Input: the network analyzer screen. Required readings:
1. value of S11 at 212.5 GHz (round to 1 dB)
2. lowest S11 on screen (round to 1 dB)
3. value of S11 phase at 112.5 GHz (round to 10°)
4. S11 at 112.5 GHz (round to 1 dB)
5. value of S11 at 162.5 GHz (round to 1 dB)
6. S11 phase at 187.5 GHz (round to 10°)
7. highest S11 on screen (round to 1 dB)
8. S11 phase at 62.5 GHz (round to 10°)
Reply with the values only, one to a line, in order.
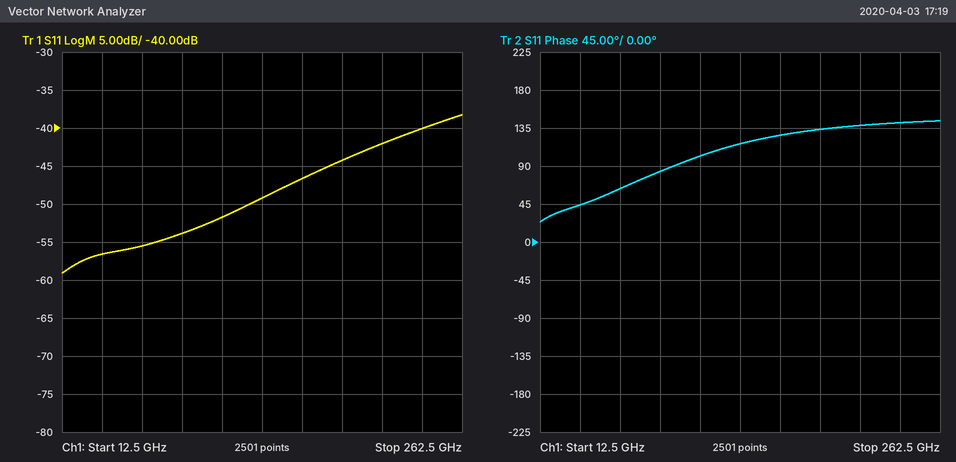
-42 dB
-59 dB
100°
-52 dB
-47 dB
130°
-38 dB
60°
